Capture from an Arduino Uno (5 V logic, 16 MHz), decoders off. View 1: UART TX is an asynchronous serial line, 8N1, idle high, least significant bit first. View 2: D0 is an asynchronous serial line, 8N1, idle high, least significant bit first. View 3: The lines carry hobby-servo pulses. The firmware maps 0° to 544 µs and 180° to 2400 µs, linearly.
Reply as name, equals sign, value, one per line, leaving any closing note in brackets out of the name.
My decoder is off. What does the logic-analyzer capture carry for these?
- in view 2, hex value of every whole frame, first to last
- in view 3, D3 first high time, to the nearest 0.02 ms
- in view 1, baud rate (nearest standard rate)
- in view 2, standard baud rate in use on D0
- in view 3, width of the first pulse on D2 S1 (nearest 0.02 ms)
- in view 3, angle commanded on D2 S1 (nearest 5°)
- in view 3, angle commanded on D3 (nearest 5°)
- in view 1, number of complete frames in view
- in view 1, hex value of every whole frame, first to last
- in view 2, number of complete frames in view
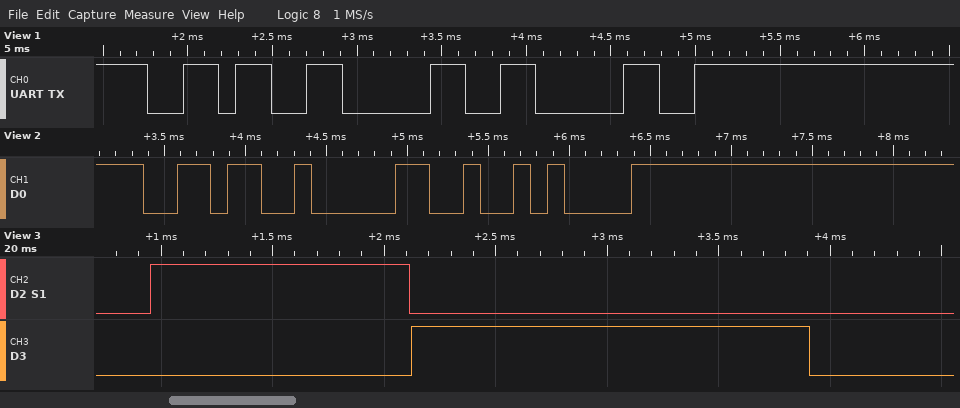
in view 2, hex value of every whole frame, first to last = 36 30 0A
in view 3, D3 first high time, to the nearest 0.02 ms = 1.78 ms
in view 1, baud rate = 9600 baud
in view 2, standard baud rate in use on D0 = 9600 baud
in view 3, width of the first pulse on D2 S1 = 1.16 ms
in view 3, angle commanded on D2 S1 = 60°
in view 3, angle commanded on D3 = 120°
in view 1, number of complete frames in view = 3
in view 1, hex value of every whole frame, first to last = 0x36 0x30 0x30
in view 2, number of complete frames in view = 3
